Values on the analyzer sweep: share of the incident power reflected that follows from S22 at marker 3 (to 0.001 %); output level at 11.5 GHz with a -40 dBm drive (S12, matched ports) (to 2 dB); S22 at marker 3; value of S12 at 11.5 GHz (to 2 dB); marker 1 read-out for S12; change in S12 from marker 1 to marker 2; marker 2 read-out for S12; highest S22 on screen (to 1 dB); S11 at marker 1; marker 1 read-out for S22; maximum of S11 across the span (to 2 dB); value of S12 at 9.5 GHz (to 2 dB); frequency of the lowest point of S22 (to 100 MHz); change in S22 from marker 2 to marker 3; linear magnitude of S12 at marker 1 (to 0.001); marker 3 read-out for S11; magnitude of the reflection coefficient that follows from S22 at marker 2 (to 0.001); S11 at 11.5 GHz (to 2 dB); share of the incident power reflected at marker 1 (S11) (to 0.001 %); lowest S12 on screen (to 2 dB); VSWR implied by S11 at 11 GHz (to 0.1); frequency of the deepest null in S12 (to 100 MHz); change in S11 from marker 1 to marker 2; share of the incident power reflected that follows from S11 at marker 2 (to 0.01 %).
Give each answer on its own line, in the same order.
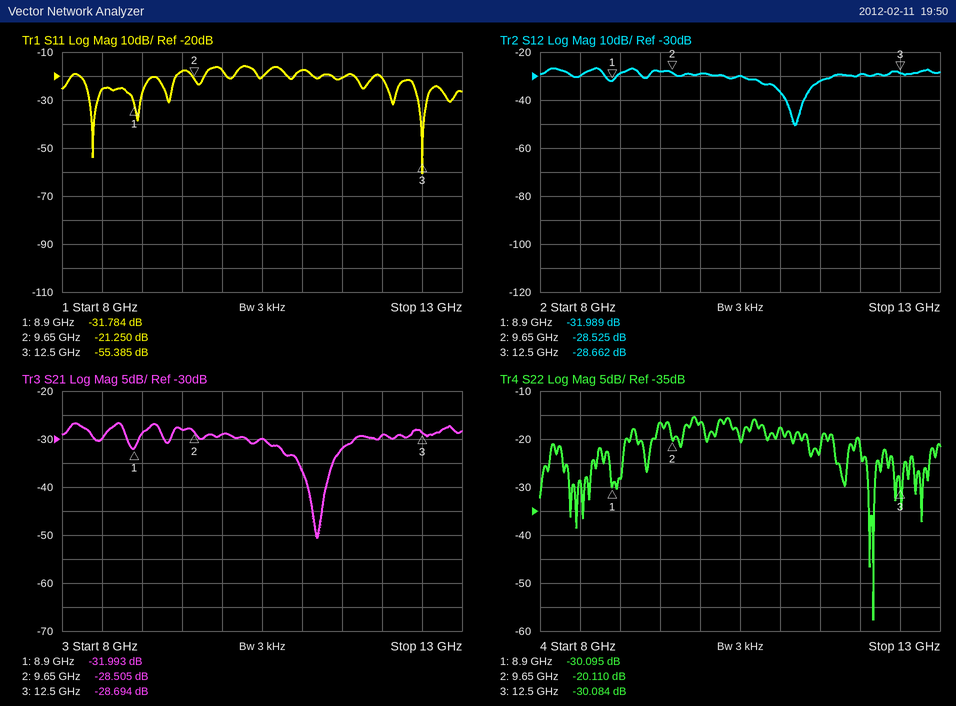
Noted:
0.098 %
-72 dBm
-30.084 dB
-32 dB
-31.989 dB
3.464 dB
-28.525 dB
-15 dB
-31.784 dB
-30.095 dB
-16 dB
-28 dB
12.2 GHz
-9.974 dB
0.025
-55.385 dB
0.099
-20 dB
0.066 %
-50 dB
1.3
11.2 GHz
10.534 dB
0.75 %
